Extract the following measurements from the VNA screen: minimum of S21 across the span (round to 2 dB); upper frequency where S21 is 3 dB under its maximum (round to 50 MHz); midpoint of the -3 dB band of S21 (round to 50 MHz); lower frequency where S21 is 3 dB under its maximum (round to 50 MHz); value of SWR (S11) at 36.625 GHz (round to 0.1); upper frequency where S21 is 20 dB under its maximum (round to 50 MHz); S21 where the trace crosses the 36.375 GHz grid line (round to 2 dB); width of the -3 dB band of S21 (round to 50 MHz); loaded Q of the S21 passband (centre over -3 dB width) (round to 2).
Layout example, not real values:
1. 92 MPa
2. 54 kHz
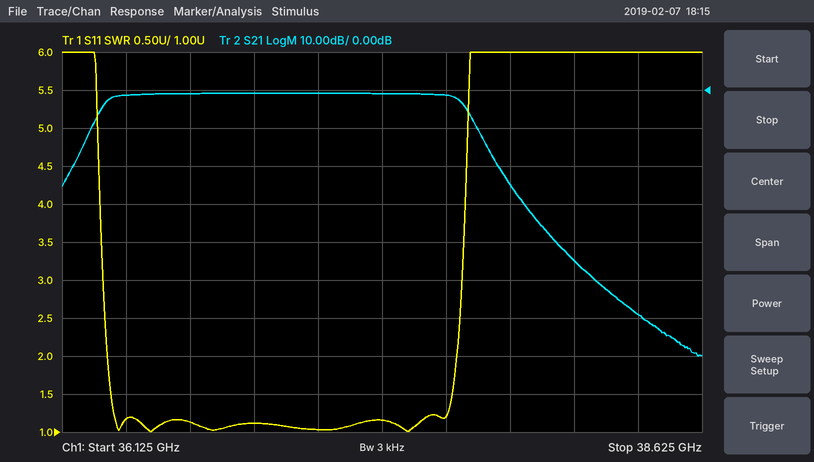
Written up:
1. -70 dB
2. 37.70 GHz
3. 37.00 GHz
4. 36.30 GHz
5. 1.1
6. 37.85 GHz
7. -2 dB
8. 1.40 GHz
9. 26
